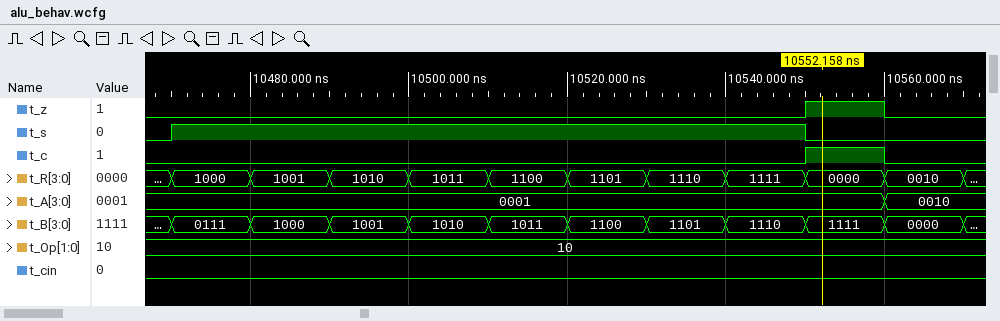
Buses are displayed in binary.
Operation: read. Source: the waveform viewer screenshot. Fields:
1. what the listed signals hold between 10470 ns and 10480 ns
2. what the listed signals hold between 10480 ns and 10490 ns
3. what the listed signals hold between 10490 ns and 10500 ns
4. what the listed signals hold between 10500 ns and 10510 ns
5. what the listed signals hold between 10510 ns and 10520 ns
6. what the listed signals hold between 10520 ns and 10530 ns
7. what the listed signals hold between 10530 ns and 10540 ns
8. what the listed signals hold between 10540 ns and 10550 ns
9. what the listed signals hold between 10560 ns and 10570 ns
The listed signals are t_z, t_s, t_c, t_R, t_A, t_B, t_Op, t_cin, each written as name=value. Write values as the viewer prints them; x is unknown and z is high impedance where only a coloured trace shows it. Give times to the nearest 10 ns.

t_z=0, t_s=1, t_c=0, t_R=1000, t_A=0001, t_B=0111, t_Op=10, t_cin=0
t_z=0, t_s=1, t_c=0, t_R=1001, t_A=0001, t_B=1000, t_Op=10, t_cin=0
t_z=0, t_s=1, t_c=0, t_R=1010, t_A=0001, t_B=1001, t_Op=10, t_cin=0
t_z=0, t_s=1, t_c=0, t_R=1011, t_A=0001, t_B=1010, t_Op=10, t_cin=0
t_z=0, t_s=1, t_c=0, t_R=1100, t_A=0001, t_B=1011, t_Op=10, t_cin=0
t_z=0, t_s=1, t_c=0, t_R=1101, t_A=0001, t_B=1100, t_Op=10, t_cin=0
t_z=0, t_s=1, t_c=0, t_R=1110, t_A=0001, t_B=1101, t_Op=10, t_cin=0
t_z=0, t_s=1, t_c=0, t_R=1111, t_A=0001, t_B=1110, t_Op=10, t_cin=0
t_z=0, t_s=0, t_c=0, t_R=0010, t_A=0010, t_B=0000, t_Op=10, t_cin=0
